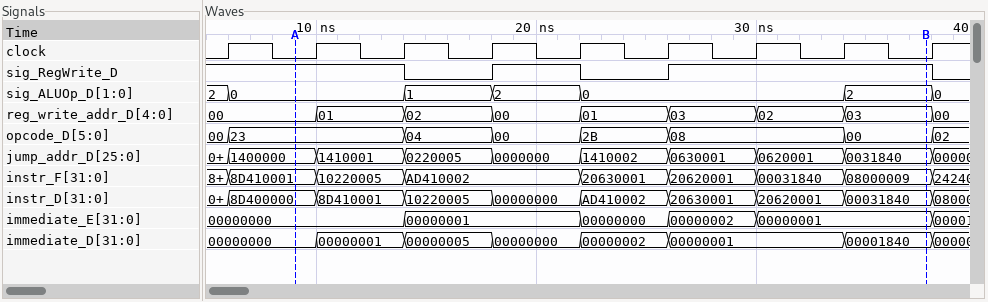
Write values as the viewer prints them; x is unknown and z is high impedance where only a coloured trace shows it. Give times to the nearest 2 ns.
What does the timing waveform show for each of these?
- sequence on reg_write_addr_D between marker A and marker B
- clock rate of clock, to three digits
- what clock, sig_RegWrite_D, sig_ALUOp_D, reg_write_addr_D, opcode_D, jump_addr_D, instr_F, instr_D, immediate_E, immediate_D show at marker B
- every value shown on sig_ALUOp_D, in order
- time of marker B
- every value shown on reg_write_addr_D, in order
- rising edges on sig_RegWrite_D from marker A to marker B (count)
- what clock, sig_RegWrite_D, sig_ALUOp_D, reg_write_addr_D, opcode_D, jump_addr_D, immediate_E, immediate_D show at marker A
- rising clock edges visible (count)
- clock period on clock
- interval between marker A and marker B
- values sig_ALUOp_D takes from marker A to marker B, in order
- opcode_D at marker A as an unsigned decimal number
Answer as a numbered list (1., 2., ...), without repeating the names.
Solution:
1. 00, 01, 02, 00, 01, 03, 02, 03
2. 250 MHz
3. clock=0, sig_RegWrite_D=1, sig_ALUOp_D=2, reg_write_addr_D=03, opcode_D=00, jump_addr_D=0031840, instr_F=08000009, instr_D=00031840, immediate_E=00000001, immediate_D=00001840
4. 2, 0, 1, 2, 0, 2, 0
5. 38 ns
6. 00, 01, 02, 00, 01, 03, 02, 03, 00
7. 2
8. clock=0, sig_RegWrite_D=1, sig_ALUOp_D=0, reg_write_addr_D=00, opcode_D=23, jump_addr_D=1400000, immediate_E=00000000, immediate_D=00000000
9. 9
10. 4 ns
11. 28 ns
12. 0, 1, 2, 0, 2
13. 35
